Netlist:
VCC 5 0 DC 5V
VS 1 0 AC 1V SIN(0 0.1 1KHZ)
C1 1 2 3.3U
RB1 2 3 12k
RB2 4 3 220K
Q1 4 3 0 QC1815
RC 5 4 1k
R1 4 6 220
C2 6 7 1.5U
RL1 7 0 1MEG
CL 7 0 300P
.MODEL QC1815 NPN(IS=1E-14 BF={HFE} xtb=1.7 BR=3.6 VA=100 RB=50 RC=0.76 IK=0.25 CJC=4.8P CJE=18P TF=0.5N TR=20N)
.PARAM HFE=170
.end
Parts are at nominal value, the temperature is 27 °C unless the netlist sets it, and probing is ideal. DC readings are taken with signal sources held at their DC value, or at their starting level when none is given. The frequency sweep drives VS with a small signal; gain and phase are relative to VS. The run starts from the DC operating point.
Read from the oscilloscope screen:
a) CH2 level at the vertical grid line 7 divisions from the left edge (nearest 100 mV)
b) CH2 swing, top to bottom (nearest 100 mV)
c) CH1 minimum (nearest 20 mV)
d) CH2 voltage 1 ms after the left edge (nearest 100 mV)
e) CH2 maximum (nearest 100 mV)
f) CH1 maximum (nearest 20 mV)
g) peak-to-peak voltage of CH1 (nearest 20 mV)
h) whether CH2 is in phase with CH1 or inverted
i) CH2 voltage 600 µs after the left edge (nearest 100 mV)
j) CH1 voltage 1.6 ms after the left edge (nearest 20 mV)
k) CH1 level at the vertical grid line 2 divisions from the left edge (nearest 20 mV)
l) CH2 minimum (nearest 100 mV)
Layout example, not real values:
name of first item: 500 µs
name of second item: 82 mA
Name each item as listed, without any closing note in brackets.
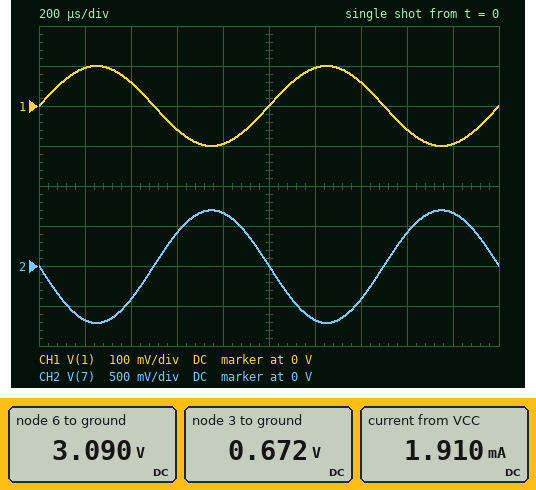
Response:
CH2 level at the vertical grid line 7 divisions from the left edge: -400 mV
CH2 swing, top to bottom: 1.4 V
CH1 minimum: -100 mV
CH2 voltage 1 ms after the left edge: 0 V
CH2 maximum: 700 mV
CH1 maximum: 100 mV
peak-to-peak voltage of CH1: 200 mV
whether CH2 is in phase with CH1 or inverted: inverted
CH2 voltage 600 µs after the left edge: 400 mV
CH1 voltage 1.6 ms after the left edge: -60 mV
CH1 level at the vertical grid line 2 divisions from the left edge: 60 mV
CH2 minimum: -700 mV
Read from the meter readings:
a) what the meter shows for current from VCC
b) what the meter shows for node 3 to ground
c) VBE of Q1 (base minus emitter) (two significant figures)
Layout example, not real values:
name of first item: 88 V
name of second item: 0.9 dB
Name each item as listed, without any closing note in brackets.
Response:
what the meter shows for current from VCC: 1.910 mA
what the meter shows for node 3 to ground: 0.672 V
VBE of Q1 (base minus emitter): 670 mV
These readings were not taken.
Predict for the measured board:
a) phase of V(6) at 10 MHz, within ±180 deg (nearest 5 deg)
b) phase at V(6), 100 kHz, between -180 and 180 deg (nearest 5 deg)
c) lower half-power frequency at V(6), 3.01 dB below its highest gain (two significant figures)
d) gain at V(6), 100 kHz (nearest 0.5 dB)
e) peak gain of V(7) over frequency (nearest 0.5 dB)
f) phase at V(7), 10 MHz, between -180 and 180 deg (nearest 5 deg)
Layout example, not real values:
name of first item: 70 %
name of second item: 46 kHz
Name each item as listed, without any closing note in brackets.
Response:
phase of V(6) at 10 MHz, within ±180 deg: 10 deg
phase at V(6), 100 kHz, between -180 and 180 deg: 160 deg
lower half-power frequency at V(6), 3.01 dB below its highest gain: 3.6 Hz
gain at V(6), 100 kHz: 16.5 dB
peak gain of V(7) over frequency: 17.0 dB
phase at V(7), 10 MHz, between -180 and 180 deg: 10 deg
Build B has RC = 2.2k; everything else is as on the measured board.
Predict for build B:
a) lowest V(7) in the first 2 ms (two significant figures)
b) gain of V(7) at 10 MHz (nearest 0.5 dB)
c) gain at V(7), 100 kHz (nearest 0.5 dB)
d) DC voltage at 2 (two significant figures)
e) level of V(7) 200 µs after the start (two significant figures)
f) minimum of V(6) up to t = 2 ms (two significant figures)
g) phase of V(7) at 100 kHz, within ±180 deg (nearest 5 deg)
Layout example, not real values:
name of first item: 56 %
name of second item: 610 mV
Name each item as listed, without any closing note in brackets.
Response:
lowest V(7) in the first 2 ms: -1.0 V
gain of V(7) at 10 MHz: -29.5 dB
gain at V(7), 100 kHz: 19.5 dB
DC voltage at 2: 660 mV
level of V(7) 200 µs after the start: -970 mV
minimum of V(6) up to t = 2 ms: 1.2 V
phase of V(7) at 100 kHz, within ±180 deg: 150 deg
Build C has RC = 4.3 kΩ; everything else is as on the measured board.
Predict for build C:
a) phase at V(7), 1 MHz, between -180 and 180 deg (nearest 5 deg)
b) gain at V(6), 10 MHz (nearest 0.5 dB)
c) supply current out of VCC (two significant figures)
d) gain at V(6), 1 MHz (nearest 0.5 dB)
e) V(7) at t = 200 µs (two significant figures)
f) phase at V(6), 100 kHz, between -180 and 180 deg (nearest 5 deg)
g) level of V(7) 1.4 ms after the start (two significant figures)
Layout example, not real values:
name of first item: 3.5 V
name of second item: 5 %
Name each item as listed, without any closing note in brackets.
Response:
phase at V(7), 1 MHz, between -180 and 180 deg: 65 deg
gain at V(6), 10 MHz: -31.0 dB
supply current out of VCC: 780 µA
gain at V(6), 1 MHz: 4.5 dB
V(7) at t = 200 µs: -1.2 V
phase at V(6), 100 kHz, between -180 and 180 deg: 145 deg
level of V(7) 1.4 ms after the start: -730 mV
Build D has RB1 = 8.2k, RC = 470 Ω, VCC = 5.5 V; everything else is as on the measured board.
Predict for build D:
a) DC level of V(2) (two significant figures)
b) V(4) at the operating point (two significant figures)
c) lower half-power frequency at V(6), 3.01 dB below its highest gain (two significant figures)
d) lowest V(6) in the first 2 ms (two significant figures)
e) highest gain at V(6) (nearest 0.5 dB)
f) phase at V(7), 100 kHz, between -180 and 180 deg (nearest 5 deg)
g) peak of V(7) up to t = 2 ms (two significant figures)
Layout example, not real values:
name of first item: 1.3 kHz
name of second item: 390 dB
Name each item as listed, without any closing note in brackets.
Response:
DC level of V(2): 680 mV
V(4) at the operating point: 4.2 V
lower half-power frequency at V(6), 3.01 dB below its highest gain: 5.1 Hz
lowest V(6) in the first 2 ms: 3.6 V
highest gain at V(6): 16.0 dB
phase at V(7), 100 kHz, between -180 and 180 deg: 165 deg
peak of V(7) up to t = 2 ms: 600 mV
